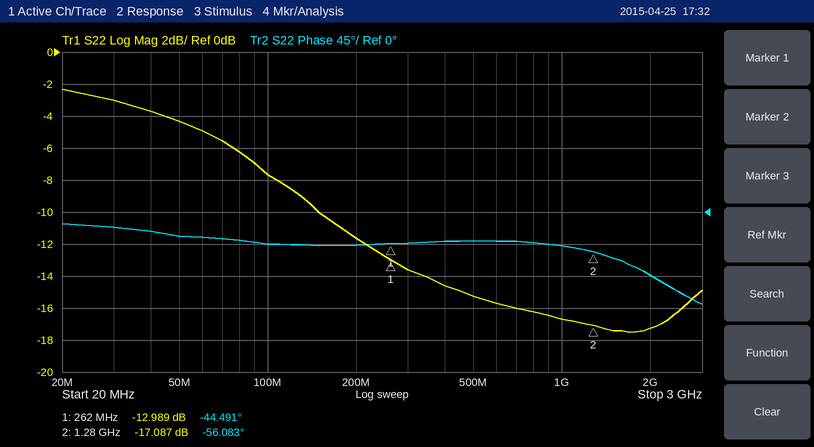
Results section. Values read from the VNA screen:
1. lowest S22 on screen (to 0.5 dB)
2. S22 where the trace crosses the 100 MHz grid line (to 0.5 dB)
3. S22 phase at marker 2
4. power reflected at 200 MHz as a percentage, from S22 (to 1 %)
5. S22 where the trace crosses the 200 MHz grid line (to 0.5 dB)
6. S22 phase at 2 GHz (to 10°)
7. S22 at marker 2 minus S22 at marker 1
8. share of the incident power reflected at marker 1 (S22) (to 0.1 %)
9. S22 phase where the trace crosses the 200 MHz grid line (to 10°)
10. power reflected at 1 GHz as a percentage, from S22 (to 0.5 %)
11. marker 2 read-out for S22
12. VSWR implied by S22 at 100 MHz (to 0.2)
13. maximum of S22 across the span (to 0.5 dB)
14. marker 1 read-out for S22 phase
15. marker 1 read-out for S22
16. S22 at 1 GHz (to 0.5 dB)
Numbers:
-17.5 dB
-7.5 dB
-56.083°
7 %
-11.5 dB
-90°
-4.098 dB
5.0 %
-50°
2.0 %
-17.087 dB
2.4
-2.5 dB
-44.491°
-12.989 dB
-16.5 dB
